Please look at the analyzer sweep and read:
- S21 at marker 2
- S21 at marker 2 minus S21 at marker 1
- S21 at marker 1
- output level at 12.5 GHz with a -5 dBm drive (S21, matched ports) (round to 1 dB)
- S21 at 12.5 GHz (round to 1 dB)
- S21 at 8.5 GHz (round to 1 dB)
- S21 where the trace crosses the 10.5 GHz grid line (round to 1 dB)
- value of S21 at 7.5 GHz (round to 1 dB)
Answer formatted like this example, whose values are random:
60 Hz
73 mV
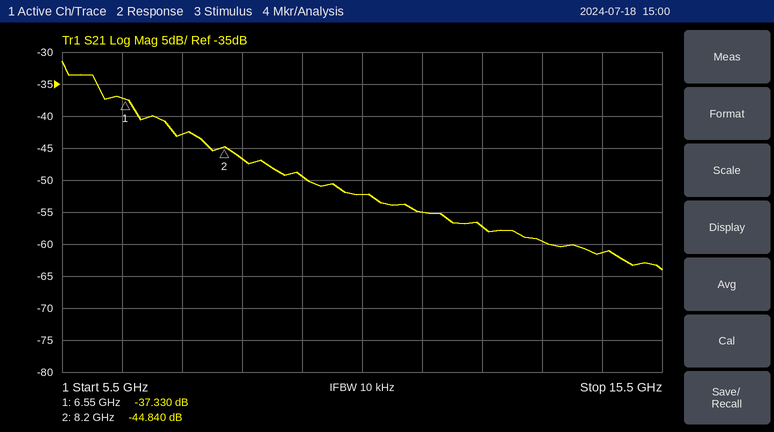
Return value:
-44.840 dB
-7.510 dB
-37.330 dB
-62 dBm
-57 dB
-47 dB
-52 dB
-43 dB
